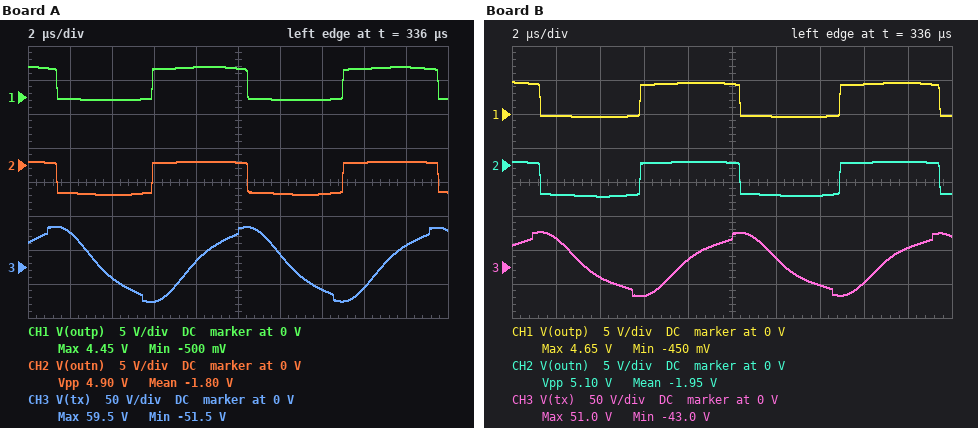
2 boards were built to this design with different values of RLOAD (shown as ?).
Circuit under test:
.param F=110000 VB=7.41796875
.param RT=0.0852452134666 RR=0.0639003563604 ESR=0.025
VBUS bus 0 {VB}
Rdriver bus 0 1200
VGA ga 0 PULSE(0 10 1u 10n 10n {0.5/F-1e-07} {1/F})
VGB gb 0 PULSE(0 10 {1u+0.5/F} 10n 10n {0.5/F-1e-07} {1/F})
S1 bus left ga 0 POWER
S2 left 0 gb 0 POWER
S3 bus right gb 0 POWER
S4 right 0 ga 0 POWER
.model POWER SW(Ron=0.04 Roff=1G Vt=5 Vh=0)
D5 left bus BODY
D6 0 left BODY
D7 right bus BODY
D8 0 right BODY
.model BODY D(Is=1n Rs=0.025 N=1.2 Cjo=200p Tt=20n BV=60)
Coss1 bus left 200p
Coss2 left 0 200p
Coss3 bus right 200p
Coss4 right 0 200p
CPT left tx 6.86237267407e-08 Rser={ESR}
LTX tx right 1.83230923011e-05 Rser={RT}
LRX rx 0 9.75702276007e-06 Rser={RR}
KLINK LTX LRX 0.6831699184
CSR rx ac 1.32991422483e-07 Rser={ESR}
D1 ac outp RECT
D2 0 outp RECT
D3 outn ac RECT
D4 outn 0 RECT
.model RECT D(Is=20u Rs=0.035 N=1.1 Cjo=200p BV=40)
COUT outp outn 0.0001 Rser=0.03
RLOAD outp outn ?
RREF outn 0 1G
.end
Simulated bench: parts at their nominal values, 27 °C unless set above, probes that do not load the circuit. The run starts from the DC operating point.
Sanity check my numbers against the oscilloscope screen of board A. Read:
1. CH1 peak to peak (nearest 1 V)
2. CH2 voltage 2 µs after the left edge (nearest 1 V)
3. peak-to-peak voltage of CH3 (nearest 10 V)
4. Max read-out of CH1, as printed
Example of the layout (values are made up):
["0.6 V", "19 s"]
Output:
["5 V", "-4 V", "110 V", "4.45 V"]
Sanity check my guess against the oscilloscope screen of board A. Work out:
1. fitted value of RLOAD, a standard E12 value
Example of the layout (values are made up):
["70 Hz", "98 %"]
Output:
["1.5 Ω"]
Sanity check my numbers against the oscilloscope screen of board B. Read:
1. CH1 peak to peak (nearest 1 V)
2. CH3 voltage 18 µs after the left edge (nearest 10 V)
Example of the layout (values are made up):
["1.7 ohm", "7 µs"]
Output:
["5 V", "30 V"]
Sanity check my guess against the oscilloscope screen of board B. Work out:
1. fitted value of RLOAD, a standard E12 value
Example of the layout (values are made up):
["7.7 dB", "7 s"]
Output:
["1.8 Ω"]
